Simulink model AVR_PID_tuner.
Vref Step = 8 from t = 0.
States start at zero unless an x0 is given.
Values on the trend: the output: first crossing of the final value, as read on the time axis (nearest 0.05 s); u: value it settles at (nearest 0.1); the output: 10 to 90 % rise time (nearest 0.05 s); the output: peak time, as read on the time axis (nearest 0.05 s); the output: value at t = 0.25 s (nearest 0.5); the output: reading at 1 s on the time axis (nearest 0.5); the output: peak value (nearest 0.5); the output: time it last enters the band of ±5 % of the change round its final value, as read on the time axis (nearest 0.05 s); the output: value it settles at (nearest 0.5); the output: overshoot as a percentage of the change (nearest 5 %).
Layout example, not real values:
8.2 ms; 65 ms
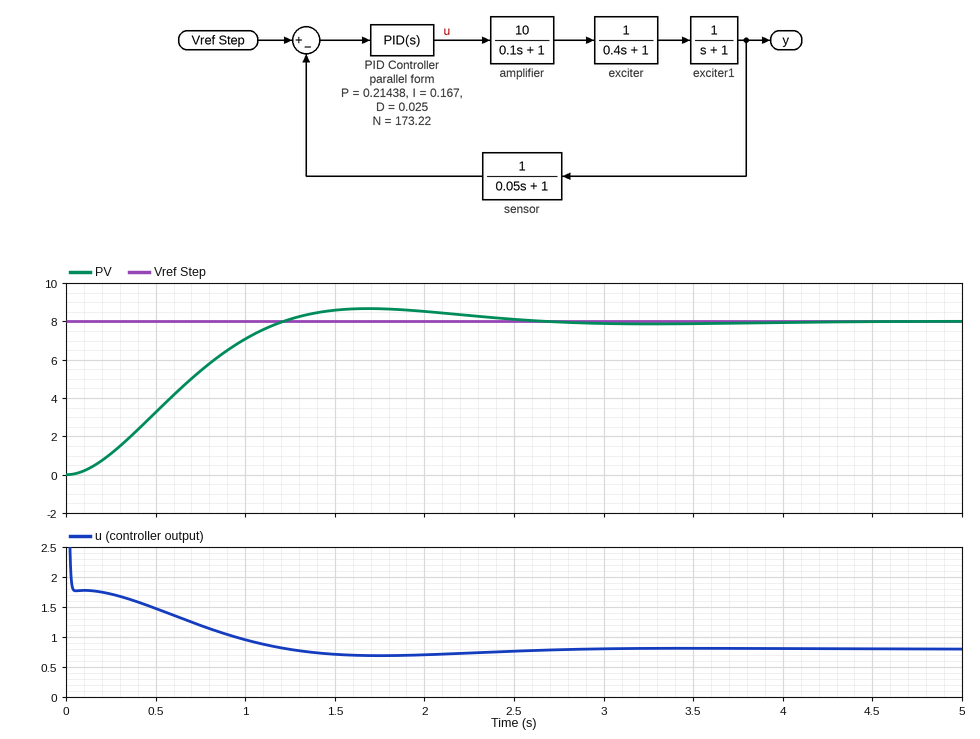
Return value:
1.20 s; 0.8; 0.80 s; 1.70 s; 1.0; 7.0; 8.5; 2.15 s; 8.0; 10 %
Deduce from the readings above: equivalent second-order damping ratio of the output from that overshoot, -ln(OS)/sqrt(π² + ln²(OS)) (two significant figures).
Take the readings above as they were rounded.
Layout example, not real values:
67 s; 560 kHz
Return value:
0.59
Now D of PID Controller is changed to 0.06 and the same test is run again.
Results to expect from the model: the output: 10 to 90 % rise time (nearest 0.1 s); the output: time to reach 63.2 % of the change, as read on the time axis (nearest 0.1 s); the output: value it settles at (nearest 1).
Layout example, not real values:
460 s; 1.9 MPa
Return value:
1.0 s; 0.6 s; 8
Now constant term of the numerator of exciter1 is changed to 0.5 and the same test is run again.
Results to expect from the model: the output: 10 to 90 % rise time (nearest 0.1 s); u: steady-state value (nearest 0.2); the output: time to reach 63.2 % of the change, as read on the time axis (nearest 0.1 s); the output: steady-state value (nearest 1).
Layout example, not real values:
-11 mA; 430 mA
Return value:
1.8 s; 1.6; 1.2 s; 8
